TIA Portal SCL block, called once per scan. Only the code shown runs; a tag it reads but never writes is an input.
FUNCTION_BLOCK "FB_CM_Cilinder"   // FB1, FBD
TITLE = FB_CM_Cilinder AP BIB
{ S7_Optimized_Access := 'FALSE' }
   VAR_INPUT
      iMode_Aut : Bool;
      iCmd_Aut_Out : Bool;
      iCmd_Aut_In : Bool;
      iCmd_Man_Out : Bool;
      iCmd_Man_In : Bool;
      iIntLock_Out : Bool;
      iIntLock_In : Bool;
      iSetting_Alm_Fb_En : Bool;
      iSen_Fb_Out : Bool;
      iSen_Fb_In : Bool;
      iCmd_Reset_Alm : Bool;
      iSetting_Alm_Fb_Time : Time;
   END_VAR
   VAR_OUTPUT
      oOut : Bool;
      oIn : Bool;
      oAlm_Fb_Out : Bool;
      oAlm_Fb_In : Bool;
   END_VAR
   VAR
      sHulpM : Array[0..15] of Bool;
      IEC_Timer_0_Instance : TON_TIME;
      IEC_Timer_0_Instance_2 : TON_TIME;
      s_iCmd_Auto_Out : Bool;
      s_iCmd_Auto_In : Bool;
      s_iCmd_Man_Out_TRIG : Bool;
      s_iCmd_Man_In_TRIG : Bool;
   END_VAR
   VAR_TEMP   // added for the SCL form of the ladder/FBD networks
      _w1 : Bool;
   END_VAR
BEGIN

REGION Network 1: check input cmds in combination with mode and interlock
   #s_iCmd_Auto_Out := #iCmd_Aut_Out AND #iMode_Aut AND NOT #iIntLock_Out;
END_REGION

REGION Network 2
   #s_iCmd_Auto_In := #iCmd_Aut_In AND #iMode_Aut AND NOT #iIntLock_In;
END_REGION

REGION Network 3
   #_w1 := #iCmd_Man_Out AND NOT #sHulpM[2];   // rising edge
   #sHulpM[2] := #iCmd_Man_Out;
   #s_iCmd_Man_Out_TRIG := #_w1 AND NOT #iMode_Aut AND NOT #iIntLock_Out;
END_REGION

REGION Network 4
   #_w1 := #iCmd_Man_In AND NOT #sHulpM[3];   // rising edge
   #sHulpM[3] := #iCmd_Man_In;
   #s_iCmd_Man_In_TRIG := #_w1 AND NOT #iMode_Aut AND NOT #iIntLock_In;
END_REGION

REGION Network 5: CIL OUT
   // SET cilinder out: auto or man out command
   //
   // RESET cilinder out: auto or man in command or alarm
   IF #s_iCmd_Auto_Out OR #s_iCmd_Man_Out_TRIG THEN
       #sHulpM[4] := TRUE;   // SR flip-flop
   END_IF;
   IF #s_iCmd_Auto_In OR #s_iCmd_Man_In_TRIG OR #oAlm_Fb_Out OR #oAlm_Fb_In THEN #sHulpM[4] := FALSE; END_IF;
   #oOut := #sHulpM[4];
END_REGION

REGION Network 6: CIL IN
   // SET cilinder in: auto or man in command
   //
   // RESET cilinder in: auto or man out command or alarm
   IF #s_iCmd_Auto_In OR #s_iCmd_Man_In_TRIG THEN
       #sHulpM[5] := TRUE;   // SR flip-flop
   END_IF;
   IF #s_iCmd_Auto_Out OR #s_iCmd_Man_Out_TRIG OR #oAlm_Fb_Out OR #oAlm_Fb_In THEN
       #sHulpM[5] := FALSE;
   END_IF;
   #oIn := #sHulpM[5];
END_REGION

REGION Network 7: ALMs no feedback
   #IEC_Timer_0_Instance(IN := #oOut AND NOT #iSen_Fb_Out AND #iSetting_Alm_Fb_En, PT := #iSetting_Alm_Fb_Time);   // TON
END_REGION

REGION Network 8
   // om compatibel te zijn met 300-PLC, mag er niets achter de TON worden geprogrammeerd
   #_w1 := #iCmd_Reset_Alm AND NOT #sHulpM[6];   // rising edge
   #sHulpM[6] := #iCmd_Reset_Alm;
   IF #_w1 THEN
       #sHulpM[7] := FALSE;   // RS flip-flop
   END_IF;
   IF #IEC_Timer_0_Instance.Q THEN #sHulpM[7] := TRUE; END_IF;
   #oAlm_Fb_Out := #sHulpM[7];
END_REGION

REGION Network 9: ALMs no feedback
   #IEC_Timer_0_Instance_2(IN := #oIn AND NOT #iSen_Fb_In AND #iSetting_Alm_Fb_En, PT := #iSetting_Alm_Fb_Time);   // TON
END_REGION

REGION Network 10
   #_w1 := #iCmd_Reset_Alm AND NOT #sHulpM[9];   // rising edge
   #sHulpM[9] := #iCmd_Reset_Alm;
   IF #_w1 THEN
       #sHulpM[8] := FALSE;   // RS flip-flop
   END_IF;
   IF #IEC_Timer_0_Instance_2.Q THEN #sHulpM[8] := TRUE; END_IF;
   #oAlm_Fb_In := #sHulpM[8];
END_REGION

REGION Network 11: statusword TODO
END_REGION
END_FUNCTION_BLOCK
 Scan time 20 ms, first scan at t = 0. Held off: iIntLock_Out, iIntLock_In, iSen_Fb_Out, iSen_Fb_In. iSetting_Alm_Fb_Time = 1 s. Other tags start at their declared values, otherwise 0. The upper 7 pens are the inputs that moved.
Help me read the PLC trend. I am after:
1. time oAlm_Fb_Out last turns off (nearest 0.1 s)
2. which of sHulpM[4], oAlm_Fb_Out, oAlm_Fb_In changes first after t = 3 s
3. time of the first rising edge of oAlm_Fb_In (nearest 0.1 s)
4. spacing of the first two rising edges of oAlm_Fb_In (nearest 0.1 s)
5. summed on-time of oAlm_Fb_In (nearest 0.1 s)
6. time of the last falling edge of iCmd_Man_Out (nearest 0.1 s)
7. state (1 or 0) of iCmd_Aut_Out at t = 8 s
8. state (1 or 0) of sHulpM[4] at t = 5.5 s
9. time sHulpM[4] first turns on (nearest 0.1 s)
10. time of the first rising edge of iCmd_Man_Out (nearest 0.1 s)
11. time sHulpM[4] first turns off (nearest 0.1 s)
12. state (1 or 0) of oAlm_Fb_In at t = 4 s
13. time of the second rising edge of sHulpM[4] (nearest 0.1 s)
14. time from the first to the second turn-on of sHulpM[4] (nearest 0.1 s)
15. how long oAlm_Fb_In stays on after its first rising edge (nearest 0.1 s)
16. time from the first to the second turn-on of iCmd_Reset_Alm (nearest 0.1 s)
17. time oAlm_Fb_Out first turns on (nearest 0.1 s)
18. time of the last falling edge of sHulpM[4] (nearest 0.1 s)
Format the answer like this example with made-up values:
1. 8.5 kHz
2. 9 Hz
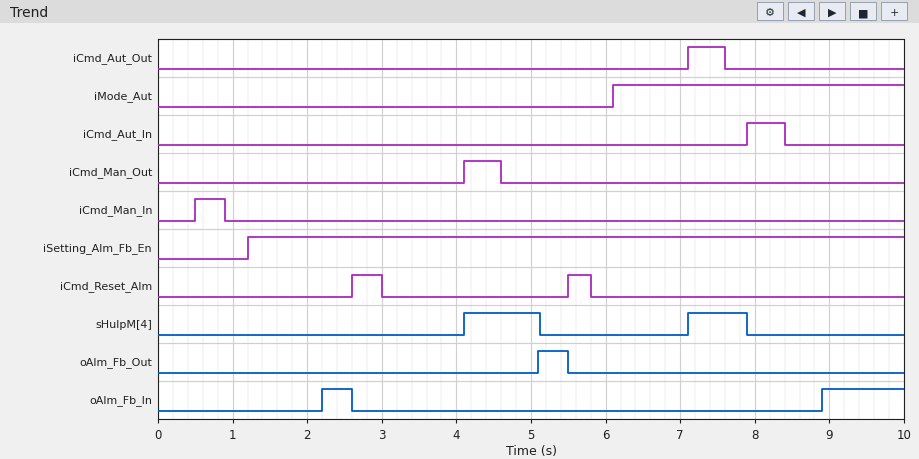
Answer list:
1. 5.5 s
2. sHulpM[4]
3. 2.2 s
4. 6.7 s
5. 1.5 s
6. 4.6 s
7. 0
8. 0
9. 4.1 s
10. 4.1 s
11. 5.1 s
12. 0
13. 7.1 s
14. 3.0 s
15. 0.4 s
16. 2.9 s
17. 5.1 s
18. 7.9 s
